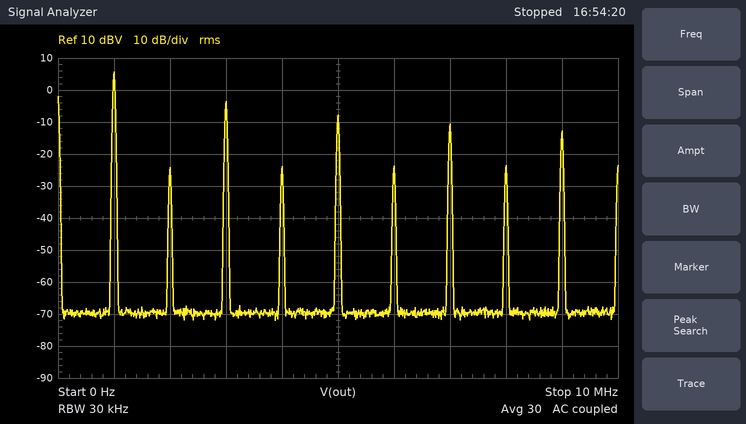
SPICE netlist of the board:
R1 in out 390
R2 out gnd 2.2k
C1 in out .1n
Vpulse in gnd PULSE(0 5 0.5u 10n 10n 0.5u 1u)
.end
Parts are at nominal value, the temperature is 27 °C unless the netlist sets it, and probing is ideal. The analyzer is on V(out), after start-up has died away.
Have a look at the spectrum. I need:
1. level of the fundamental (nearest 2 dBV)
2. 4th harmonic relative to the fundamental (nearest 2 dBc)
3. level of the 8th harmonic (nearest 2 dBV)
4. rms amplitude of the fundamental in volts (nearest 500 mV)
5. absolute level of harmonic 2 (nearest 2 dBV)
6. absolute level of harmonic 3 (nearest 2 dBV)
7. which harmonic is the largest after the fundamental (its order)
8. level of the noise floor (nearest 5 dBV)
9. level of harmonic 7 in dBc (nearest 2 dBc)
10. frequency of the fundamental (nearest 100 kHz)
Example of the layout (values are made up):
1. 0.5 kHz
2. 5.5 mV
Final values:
1. 6 dBV
2. -30 dBc
3. -24 dBV
4. 2.0 V
5. -24 dBV
6. -4 dBV
7. 3
8. -70 dBV
9. -16 dBc
10. 1.0 MHz
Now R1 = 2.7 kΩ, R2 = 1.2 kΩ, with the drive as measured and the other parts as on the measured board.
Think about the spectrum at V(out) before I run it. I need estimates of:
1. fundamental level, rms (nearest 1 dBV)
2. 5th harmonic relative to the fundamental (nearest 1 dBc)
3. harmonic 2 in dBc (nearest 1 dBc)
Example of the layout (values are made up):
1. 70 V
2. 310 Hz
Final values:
1. 2 dBV
2. -9 dBc
3. -27 dBc
